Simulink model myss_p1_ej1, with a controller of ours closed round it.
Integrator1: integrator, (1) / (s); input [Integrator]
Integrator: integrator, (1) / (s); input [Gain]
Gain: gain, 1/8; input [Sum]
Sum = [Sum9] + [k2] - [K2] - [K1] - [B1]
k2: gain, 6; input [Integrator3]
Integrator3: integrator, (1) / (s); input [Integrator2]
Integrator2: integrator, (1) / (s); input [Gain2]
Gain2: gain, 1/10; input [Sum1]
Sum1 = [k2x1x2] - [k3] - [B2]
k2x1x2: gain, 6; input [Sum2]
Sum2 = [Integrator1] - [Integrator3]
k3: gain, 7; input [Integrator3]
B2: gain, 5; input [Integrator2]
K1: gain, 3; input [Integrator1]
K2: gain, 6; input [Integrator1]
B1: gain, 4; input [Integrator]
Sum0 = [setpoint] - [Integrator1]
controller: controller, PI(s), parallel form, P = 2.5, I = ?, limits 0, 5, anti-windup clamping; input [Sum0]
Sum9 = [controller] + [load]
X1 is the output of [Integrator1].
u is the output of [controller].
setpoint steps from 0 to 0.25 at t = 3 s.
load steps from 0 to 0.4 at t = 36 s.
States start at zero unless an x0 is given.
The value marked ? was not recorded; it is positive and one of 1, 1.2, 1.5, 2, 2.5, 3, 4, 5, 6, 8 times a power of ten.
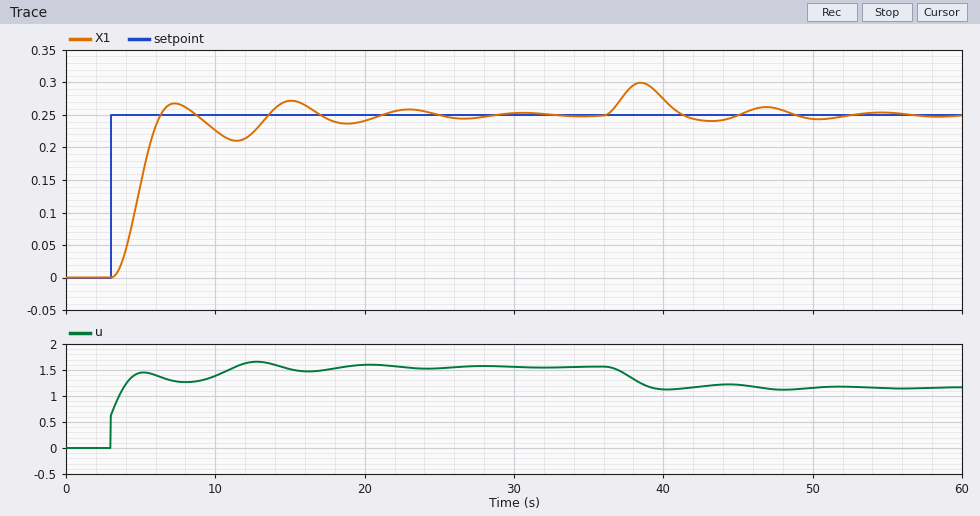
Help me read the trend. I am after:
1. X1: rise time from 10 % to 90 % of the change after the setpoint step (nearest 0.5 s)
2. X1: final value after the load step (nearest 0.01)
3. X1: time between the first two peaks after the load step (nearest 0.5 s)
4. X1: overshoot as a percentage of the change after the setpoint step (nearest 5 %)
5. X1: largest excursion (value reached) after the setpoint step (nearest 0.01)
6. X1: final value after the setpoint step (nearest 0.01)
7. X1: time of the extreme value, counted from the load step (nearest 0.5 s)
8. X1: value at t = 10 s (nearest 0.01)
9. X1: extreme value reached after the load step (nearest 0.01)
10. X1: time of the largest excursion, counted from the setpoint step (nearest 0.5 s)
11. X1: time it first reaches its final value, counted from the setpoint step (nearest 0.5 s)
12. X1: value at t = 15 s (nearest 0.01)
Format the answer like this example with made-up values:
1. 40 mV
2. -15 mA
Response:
1. 2.0 s
2. 0.25
3. 8.5 s
4. 10 %
5. 0.27
6. 0.25
7. 2.5 s
8. 0.23
9. 0.30
10. 12.0 s
11. 3.5 s
12. 0.27
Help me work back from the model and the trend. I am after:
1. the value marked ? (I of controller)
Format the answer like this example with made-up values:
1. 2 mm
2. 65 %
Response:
1. 3
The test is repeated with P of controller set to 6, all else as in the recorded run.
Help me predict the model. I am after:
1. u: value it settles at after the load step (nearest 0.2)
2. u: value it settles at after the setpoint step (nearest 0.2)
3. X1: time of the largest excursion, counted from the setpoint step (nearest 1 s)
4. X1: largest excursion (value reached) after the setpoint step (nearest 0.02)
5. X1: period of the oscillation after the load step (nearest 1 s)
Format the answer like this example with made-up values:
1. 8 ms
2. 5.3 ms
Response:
1. 1.2
2. 1.6
3. 11 s
4. 0.26
5. 8 s
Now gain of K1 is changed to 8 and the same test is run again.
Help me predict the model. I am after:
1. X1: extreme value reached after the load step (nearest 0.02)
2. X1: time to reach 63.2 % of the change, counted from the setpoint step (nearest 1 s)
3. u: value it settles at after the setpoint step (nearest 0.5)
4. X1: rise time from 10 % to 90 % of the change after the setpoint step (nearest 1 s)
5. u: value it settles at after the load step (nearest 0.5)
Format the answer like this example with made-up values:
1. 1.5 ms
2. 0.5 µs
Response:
1. 0.28
2. 3 s
3. 3.0
4. 9 s
5. 2.5
